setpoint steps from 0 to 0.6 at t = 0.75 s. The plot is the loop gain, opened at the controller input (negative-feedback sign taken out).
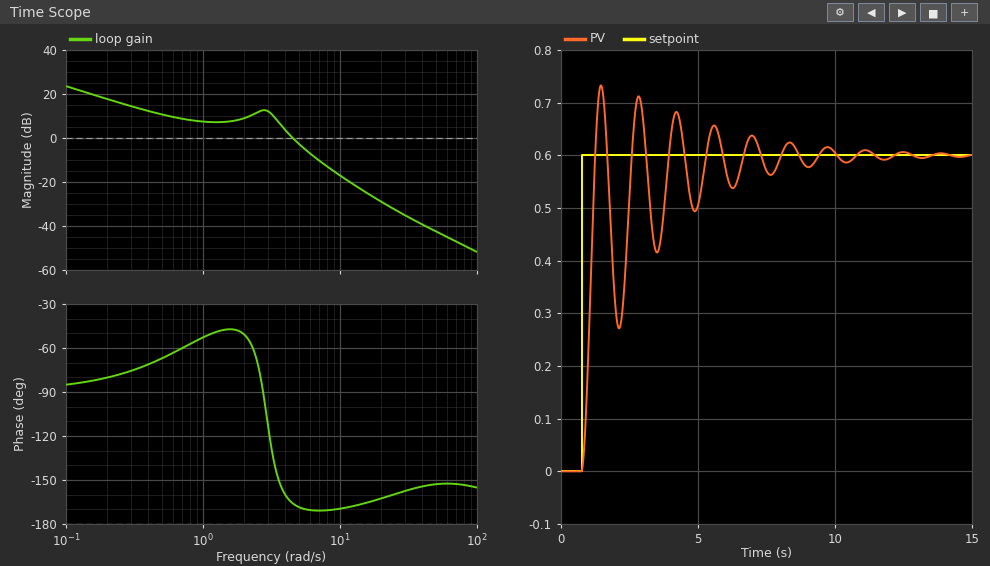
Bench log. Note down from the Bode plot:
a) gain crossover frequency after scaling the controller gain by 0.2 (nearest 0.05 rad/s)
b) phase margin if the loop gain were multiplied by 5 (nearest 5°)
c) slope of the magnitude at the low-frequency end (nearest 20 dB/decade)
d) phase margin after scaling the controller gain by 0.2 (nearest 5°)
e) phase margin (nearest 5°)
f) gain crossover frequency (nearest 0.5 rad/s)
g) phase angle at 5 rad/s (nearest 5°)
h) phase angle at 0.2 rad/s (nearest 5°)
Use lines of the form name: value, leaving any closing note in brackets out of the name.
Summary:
gain crossover frequency after scaling the controller gain by 0.2: 0.30 rad/s
phase margin if the loop gain were multiplied by 5: 10°
slope of the magnitude at the low-frequency end: -20 dB/decade
phase margin after scaling the controller gain by 0.2: 105°
phase margin: 15°
gain crossover frequency: 4.5 rad/s
phase angle at 5 rad/s: -170°
phase angle at 0.2 rad/s: -80°
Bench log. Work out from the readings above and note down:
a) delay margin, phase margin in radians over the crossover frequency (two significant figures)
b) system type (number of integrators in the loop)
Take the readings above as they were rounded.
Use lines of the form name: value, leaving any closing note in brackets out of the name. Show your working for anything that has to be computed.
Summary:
delay margin, phase margin in radians over the crossover frequency: 15 × π / 180 / 4.5 = 0.058 s
system type: 1
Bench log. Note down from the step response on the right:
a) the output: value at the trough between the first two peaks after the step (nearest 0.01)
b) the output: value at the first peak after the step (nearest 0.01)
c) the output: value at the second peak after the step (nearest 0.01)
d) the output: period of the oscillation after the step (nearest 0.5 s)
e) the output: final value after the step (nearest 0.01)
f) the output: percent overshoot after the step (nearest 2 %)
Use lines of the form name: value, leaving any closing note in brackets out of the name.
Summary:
the output: value at the trough between the first two peaks after the step: 0.27
the output: value at the first peak after the step: 0.73
the output: value at the second peak after the step: 0.71
the output: period of the oscillation after the step: 1.5 s
the output: final value after the step: 0.60
the output: percent overshoot after the step: 22 %
